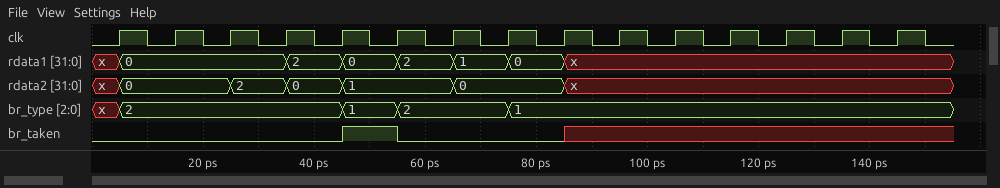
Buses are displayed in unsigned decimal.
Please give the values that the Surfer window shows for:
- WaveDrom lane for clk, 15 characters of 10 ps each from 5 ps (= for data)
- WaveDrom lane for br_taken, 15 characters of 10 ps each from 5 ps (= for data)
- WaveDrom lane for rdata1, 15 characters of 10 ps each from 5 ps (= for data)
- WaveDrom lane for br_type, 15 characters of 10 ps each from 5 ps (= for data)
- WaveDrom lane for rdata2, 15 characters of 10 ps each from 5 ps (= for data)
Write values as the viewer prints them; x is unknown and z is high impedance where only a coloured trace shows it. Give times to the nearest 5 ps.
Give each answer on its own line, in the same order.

{name: 'clk', wave: 'p..............'}
{name: 'br_taken', wave: '0...10..x......'}
{name: 'rdata1', wave: '=..=====x......', data: '0 2 0 2 1 0'}
{name: 'br_type', wave: '=...==.=.......', data: '2 1 2 1'}
{name: 'rdata2', wave: '=.===.=.x......', data: '0 2 0 1 0'}
